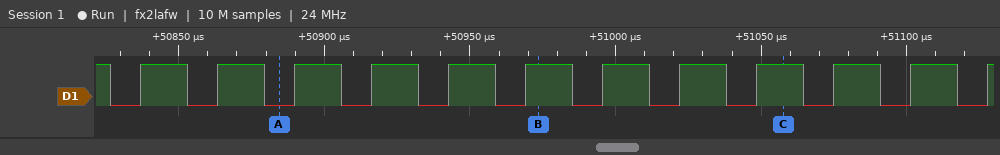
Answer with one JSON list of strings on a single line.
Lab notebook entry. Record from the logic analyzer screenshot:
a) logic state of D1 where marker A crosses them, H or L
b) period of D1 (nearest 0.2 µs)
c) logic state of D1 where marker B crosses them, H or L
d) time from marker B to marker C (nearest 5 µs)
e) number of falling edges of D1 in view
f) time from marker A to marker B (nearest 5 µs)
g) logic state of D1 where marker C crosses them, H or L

["D1=L", "26.4 µs", "D1=H", "85 µs", "12", "90 µs", "D1=H"]
